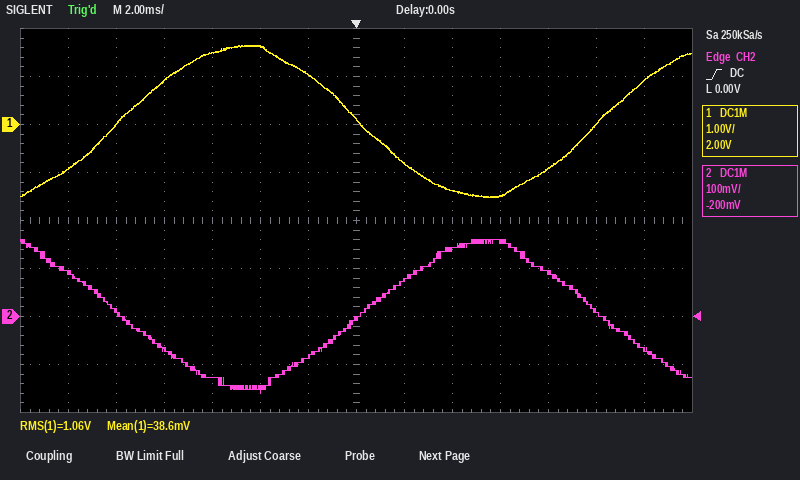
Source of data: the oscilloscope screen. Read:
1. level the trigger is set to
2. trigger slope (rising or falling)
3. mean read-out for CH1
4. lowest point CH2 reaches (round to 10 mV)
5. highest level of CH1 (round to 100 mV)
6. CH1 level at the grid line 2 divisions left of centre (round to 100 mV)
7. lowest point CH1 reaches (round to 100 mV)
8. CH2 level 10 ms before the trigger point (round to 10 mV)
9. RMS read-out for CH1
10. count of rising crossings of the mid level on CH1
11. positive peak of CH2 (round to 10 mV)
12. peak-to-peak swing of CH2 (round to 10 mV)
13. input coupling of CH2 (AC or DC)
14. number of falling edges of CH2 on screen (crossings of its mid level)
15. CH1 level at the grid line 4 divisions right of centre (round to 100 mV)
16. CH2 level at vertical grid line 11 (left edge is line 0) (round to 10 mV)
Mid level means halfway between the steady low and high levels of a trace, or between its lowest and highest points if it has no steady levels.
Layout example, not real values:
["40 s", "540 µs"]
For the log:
["0.00 V", "rising", "38.6 mV", "-160 mV", "1.6 V", "1.6 V", "-1.5 V", "10 mV", "1.06 V", "2", "160 mV", "320 mV", "DC", "2", "-900 mV", "90 mV"]
